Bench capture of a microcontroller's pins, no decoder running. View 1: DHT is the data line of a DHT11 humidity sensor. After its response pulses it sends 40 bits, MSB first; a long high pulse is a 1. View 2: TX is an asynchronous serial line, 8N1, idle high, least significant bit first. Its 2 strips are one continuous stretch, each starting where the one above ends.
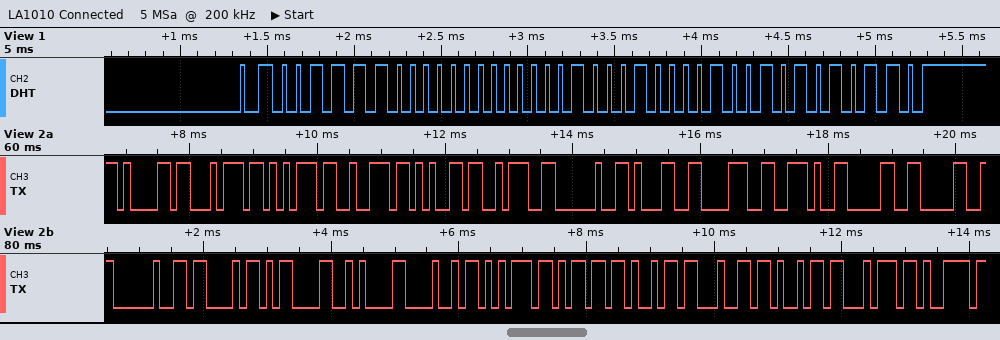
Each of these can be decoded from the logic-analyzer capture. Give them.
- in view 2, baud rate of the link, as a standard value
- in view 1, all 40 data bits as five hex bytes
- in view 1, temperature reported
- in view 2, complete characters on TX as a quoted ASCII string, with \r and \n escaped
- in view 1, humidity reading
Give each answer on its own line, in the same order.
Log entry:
9600 baud
3C 00 11 09 56
17.9 °C
"ature: 18.00 C\r\nHumidity"
60 %
